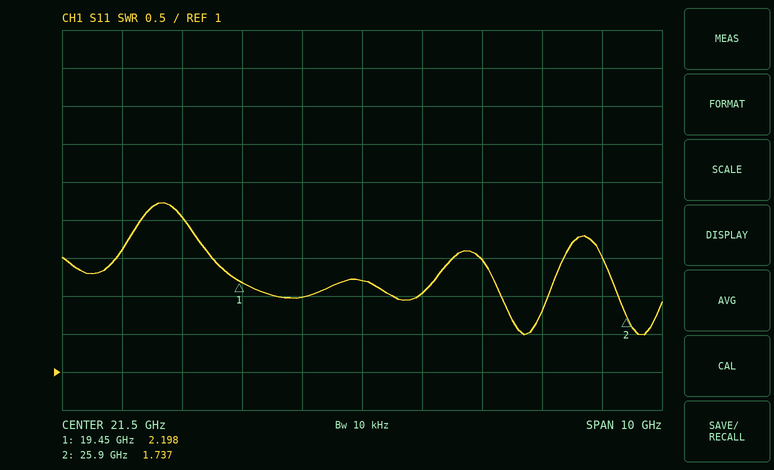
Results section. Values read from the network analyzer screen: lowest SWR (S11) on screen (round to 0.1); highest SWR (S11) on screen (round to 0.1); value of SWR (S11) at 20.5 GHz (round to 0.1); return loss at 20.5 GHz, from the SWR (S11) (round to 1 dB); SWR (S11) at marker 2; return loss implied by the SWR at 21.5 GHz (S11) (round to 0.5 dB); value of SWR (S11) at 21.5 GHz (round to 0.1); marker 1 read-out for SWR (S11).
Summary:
1.5
3.2
2.0
10 dB
1.737
8.5 dB
2.2
2.198
